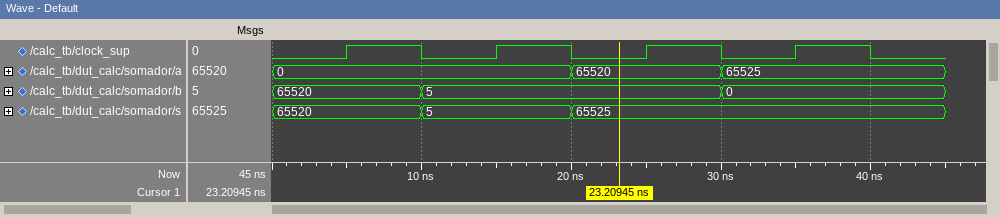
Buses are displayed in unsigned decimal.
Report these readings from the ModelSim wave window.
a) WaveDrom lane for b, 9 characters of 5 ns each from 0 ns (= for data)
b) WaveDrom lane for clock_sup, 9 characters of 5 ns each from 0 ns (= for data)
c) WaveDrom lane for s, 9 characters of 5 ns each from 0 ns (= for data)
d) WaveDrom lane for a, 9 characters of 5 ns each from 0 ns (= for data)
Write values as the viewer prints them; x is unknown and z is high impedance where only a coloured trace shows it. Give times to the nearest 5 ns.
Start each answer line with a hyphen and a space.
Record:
- {name: 'b', wave: '=.=...=..', data: '65520 5 0'}
- {name: 'clock_sup', wave: '010101010'}
- {name: 's', wave: '=.=.=....', data: '65520 5 65525'}
- {name: 'a', wave: '=...=.=..', data: '0 65520 65525'}
